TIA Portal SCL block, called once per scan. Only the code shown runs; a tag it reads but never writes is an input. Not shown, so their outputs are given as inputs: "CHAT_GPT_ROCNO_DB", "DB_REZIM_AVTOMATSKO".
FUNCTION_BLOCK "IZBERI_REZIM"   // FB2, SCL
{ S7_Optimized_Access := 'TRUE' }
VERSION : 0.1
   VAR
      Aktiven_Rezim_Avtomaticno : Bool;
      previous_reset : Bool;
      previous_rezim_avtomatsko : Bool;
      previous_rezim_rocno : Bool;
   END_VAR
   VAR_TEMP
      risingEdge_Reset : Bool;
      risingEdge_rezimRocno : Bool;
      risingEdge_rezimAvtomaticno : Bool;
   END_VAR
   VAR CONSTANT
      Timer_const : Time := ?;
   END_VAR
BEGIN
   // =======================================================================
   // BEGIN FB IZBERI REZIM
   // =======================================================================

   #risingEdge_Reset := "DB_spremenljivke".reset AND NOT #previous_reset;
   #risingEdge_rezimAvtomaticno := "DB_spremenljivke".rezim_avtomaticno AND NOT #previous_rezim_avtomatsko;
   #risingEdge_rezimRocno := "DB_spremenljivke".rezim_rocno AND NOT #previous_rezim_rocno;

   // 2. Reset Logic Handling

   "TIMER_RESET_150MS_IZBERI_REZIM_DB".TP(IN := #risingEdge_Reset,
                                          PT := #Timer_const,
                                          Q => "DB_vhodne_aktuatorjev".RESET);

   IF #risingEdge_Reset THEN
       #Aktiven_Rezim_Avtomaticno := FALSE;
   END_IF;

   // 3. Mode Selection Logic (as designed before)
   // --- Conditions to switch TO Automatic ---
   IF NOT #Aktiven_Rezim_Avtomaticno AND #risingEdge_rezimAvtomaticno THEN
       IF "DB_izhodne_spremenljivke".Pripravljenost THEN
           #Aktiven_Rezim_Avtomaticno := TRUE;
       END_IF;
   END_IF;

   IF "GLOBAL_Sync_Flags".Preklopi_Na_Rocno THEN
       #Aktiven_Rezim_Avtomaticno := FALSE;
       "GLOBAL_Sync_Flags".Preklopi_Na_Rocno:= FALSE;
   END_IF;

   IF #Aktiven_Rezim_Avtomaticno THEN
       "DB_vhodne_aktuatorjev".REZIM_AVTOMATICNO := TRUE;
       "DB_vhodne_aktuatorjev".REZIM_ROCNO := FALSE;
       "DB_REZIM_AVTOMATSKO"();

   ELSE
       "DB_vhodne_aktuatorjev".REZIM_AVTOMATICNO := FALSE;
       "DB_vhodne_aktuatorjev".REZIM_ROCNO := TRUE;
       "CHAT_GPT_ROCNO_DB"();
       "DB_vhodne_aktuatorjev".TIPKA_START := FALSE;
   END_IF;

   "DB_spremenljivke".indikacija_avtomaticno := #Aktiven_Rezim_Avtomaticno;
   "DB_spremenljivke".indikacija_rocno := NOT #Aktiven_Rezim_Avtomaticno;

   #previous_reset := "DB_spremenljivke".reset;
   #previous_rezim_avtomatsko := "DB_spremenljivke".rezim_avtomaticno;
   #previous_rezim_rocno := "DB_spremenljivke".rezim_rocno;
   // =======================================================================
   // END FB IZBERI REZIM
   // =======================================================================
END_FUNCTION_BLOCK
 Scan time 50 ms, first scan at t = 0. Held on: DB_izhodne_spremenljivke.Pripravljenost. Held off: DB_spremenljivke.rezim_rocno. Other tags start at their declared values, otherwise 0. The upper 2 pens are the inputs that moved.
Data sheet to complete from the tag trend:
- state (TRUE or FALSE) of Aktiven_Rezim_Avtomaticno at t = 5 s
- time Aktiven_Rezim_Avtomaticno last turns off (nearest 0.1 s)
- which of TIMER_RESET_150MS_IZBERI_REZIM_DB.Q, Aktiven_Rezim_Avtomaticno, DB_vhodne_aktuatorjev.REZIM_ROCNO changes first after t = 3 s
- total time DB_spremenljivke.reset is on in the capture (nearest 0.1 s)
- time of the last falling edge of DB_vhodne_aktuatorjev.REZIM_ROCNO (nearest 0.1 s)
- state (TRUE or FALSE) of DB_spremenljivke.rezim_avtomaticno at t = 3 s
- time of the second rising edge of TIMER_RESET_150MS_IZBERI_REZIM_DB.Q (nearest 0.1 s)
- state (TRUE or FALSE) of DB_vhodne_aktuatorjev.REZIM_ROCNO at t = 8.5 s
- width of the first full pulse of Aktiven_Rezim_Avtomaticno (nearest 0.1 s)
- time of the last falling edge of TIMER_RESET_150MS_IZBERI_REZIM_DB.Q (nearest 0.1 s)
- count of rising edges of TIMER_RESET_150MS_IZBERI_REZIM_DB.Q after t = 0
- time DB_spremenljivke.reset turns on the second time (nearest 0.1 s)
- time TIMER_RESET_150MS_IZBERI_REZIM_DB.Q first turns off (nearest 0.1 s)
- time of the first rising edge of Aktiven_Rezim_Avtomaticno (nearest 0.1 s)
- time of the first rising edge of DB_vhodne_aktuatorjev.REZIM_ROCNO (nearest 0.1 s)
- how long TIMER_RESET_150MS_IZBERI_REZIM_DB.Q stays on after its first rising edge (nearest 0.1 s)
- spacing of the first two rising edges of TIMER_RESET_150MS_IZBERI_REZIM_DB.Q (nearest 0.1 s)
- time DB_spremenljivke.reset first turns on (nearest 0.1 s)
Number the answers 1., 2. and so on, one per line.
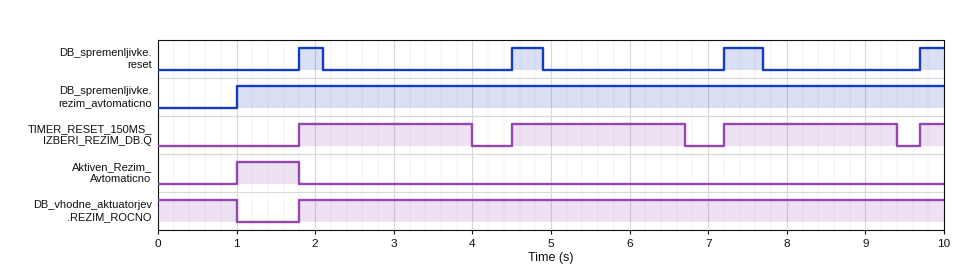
1. FALSE
2. 1.8 s
3. TIMER_RESET_150MS_IZBERI_REZIM_DB.Q
4. 1.5 s
5. 1.0 s
6. TRUE
7. 4.5 s
8. TRUE
9. 0.8 s
10. 9.4 s
11. 4
12. 4.5 s
13. 4.0 s
14. 1.0 s
15. 1.8 s
16. 2.2 s
17. 2.7 s
18. 1.8 s
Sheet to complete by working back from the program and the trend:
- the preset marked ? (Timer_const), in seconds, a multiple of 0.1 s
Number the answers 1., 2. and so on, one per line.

1. 2.2 s
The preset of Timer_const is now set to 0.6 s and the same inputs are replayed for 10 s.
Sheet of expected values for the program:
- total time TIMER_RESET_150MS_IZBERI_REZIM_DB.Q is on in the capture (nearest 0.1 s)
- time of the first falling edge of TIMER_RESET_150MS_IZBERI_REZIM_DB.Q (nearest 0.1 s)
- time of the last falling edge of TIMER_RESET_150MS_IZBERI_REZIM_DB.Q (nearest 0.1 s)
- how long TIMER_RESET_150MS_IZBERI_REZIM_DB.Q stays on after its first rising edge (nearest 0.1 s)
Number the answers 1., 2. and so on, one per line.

1. 2.1 s
2. 2.4 s
3. 7.8 s
4. 0.6 s
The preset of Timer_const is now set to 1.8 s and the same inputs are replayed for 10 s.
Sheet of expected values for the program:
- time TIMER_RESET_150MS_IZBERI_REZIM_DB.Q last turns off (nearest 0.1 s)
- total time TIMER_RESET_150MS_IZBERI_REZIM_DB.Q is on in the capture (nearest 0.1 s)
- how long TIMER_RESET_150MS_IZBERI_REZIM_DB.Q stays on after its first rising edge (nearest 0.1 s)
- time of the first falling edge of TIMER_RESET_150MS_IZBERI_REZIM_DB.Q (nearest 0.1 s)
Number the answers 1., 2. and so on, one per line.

1. 9.0 s
2. 5.7 s
3. 1.8 s
4. 3.6 s
